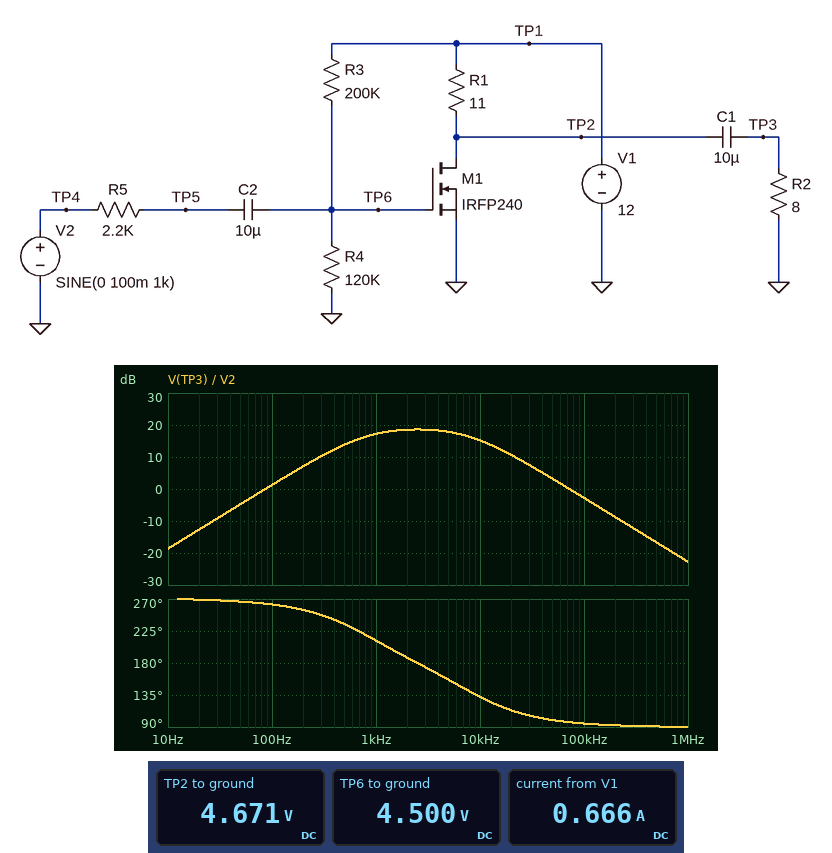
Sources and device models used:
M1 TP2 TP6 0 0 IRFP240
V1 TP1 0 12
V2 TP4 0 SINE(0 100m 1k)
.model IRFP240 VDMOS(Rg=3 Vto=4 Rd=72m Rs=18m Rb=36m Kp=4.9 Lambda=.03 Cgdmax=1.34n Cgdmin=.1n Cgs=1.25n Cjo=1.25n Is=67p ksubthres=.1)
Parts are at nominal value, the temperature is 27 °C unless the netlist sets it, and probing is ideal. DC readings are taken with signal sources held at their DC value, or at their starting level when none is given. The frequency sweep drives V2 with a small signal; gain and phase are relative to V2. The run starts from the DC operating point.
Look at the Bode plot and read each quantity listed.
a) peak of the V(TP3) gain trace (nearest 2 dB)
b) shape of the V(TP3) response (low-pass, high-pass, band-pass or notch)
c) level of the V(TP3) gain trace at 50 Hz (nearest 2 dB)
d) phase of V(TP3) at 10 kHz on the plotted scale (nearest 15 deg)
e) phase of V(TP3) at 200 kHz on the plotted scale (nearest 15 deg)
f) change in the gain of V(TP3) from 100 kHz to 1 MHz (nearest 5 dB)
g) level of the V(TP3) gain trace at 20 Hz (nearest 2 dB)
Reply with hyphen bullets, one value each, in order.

- 18 dB
- band-pass
- -4 dB
- 135 deg
- 90 deg
- -20 dB
- -12 dB
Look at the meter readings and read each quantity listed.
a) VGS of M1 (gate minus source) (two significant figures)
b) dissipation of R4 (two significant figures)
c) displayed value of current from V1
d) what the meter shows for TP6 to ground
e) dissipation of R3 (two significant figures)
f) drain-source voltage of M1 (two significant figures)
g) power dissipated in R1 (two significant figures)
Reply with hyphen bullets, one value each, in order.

- 4.5 V
- 170 µW
- 0.666 A
- 4.500 V
- 280 µW
- 4.7 V
- 4.9 W
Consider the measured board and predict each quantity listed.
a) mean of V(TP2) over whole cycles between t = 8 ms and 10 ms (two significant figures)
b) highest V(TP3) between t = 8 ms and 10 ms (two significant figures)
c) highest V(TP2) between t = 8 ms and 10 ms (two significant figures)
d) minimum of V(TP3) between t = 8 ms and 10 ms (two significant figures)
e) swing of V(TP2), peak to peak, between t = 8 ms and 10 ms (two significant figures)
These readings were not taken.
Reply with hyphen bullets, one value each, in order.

- 4.6 V
- 770 mV
- 6.2 V
- -670 mV
- 3.2 V
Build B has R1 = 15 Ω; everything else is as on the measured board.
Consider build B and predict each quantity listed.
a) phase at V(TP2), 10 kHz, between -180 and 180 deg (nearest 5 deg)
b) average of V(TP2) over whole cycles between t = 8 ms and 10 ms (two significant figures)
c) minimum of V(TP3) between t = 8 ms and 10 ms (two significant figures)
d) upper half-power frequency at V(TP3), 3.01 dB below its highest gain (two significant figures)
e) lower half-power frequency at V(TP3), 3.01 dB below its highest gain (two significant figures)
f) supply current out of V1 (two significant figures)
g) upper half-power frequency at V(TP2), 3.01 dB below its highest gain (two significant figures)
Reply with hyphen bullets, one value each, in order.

- 110 deg
- 2.5 V
- -740 mV
- 6.4 kHz
- 510 Hz
- 630 mA
- 680 Hz
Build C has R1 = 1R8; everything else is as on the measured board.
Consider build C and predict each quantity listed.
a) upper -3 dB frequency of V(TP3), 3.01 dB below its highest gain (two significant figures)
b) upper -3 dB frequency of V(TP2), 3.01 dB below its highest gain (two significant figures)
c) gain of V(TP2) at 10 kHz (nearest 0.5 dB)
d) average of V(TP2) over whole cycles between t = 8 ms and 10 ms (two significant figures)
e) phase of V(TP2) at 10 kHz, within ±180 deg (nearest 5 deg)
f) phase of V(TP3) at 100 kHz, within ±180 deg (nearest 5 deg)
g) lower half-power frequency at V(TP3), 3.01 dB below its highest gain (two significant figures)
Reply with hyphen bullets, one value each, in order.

- 38 kHz
- 20 kHz
- 12.0 dB
- 11 V
- 160 deg
- 110 deg
- 1.5 kHz
